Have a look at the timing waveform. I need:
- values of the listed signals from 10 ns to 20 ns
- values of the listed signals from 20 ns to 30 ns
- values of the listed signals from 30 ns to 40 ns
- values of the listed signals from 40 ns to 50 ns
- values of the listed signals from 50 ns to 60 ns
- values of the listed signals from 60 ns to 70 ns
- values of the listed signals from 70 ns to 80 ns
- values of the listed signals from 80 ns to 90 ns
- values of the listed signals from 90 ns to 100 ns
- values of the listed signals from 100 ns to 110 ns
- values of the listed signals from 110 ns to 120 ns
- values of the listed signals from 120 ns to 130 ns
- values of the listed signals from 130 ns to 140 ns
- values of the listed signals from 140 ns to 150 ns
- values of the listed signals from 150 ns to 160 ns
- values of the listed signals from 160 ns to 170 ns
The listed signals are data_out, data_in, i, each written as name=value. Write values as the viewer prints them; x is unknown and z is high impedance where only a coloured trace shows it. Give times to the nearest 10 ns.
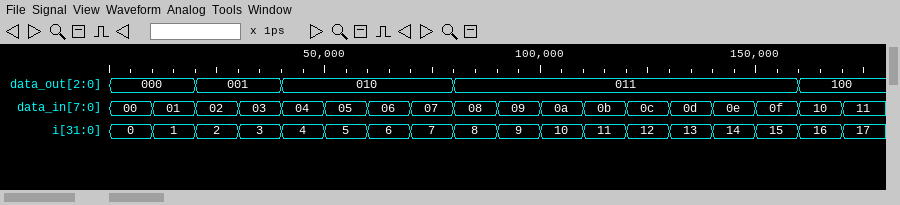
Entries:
data_out=000, data_in=01, i=1
data_out=001, data_in=02, i=2
data_out=001, data_in=03, i=3
data_out=010, data_in=04, i=4
data_out=010, data_in=05, i=5
data_out=010, data_in=06, i=6
data_out=010, data_in=07, i=7
data_out=011, data_in=08, i=8
data_out=011, data_in=09, i=9
data_out=011, data_in=0a, i=10
data_out=011, data_in=0b, i=11
data_out=011, data_in=0c, i=12
data_out=011, data_in=0d, i=13
data_out=011, data_in=0e, i=14
data_out=011, data_in=0f, i=15
data_out=100, data_in=10, i=16
